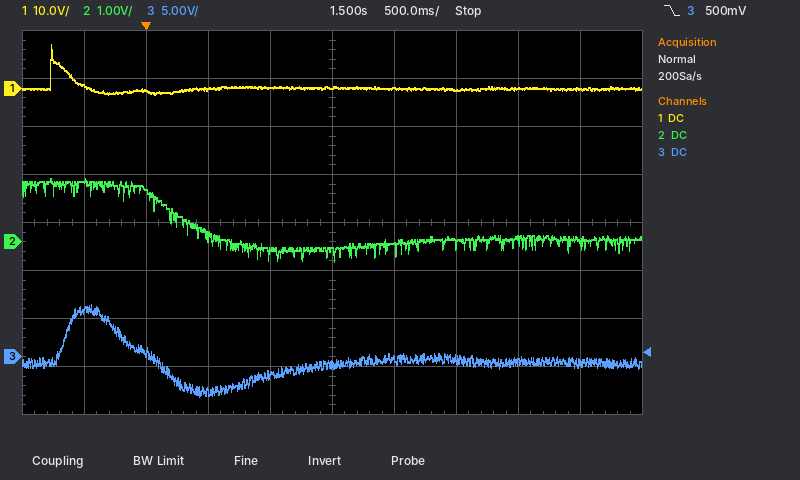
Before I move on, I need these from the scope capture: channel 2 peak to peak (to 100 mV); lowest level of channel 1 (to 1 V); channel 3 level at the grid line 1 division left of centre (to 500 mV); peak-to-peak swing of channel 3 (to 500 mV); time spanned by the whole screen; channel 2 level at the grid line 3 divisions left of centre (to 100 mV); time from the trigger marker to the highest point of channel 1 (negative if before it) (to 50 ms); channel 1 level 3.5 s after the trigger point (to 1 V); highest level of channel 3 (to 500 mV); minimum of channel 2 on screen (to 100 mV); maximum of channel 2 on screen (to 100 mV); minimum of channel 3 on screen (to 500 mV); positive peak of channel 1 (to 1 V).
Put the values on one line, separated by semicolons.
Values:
1.7 V; -1 V; -2.0 V; 9.5 V; 5 s; 1.1 V; -750 ms; 0 V; 5.5 V; -400 mV; 1.3 V; -4.0 V; 9 V
